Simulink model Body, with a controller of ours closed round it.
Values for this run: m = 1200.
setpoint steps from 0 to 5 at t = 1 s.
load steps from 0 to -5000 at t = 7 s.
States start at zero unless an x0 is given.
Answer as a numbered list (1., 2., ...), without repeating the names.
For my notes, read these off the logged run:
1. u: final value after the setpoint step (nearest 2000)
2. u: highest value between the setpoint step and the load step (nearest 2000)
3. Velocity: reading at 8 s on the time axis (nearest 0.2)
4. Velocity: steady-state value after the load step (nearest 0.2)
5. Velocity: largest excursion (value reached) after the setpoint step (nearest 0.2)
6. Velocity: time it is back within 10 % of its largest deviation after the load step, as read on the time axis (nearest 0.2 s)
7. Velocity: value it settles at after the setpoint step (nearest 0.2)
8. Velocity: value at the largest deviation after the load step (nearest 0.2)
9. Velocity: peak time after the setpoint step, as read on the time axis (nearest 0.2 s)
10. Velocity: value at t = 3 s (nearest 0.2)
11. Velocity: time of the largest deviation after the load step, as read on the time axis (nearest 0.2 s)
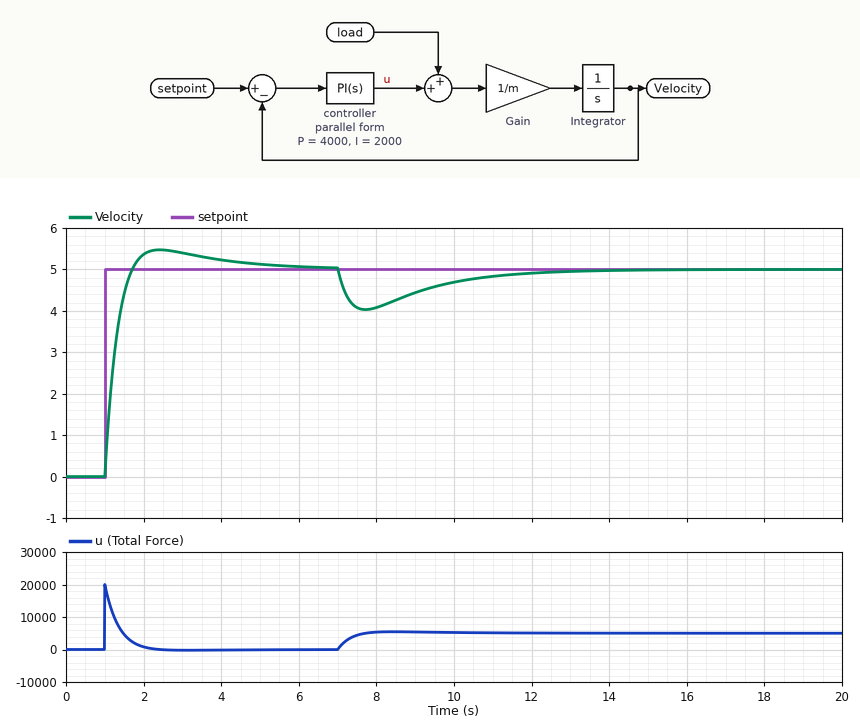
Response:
1. 0
2. 20000
3. 4.0
4. 5.0
5. 5.4
6. 11.8 s
7. 5.0
8. 4.0
9. 2.4 s
10. 5.4
11. 7.8 s
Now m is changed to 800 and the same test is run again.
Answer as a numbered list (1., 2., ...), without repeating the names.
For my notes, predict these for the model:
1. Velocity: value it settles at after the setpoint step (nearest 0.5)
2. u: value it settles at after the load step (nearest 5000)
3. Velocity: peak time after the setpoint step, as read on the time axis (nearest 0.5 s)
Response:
1. 5.0
2. 5000
3. 2.0 s
